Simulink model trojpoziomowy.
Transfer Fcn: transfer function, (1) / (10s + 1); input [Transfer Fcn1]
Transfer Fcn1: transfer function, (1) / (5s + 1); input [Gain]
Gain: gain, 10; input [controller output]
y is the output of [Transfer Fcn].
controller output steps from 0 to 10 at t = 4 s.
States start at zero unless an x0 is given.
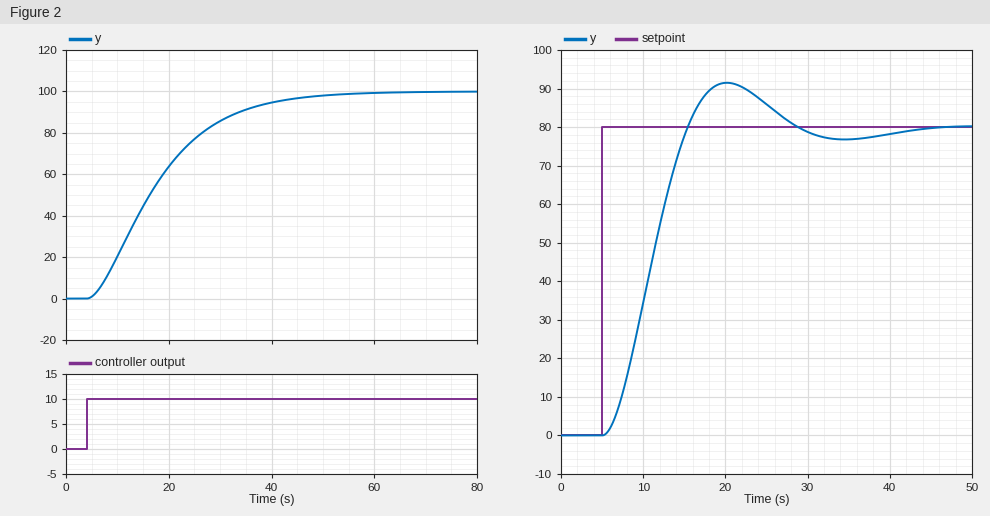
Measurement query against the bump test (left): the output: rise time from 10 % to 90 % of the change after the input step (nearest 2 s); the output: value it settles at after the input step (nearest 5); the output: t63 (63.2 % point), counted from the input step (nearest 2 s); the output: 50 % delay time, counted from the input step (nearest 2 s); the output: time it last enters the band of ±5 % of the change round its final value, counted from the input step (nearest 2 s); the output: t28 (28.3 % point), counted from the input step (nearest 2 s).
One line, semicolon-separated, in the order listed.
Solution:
26 s; 100; 16 s; 12 s; 36 s; 8 s
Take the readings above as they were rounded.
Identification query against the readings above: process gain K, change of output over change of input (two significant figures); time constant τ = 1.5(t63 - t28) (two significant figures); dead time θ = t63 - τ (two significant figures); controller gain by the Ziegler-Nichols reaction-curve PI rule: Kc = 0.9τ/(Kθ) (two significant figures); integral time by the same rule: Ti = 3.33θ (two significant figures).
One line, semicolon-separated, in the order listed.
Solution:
10; 12 s; 4.0 s; 0.27; 13 s
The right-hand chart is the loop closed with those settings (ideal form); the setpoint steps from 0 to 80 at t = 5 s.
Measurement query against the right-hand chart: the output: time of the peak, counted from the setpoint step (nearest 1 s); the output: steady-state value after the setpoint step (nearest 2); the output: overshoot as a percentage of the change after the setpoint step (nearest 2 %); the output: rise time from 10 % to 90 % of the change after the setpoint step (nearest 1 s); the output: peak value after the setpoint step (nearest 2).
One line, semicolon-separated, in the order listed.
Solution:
15 s; 80; 14 %; 7 s; 92
